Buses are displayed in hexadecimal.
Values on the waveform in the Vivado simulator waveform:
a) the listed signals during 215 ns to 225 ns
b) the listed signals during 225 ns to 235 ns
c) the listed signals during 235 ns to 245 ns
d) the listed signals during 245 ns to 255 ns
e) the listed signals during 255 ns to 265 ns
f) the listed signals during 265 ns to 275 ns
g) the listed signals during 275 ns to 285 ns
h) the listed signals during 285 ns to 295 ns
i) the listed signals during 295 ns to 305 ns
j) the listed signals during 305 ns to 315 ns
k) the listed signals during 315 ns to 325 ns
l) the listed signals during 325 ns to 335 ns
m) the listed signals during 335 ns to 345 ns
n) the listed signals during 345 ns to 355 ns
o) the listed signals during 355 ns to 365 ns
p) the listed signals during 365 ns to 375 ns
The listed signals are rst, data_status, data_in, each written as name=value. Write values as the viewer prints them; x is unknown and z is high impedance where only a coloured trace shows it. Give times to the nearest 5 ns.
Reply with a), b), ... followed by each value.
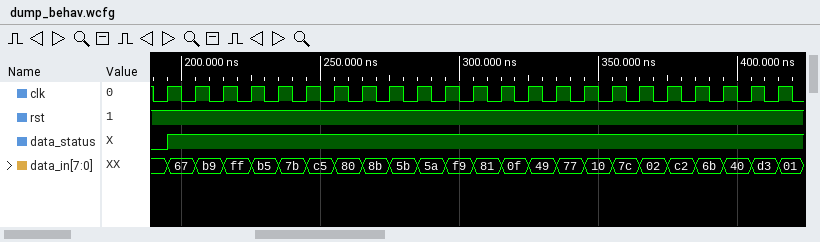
a) rst=1, data_status=1, data_in=ff
b) rst=1, data_status=1, data_in=b5
c) rst=1, data_status=1, data_in=7b
d) rst=1, data_status=1, data_in=c5
e) rst=1, data_status=1, data_in=80
f) rst=1, data_status=1, data_in=8b
g) rst=1, data_status=1, data_in=5b
h) rst=1, data_status=1, data_in=5a
i) rst=1, data_status=1, data_in=f9
j) rst=1, data_status=1, data_in=81
k) rst=1, data_status=1, data_in=0f
l) rst=1, data_status=1, data_in=49
m) rst=1, data_status=1, data_in=77
n) rst=1, data_status=1, data_in=10
o) rst=1, data_status=1, data_in=7c
p) rst=1, data_status=1, data_in=02
